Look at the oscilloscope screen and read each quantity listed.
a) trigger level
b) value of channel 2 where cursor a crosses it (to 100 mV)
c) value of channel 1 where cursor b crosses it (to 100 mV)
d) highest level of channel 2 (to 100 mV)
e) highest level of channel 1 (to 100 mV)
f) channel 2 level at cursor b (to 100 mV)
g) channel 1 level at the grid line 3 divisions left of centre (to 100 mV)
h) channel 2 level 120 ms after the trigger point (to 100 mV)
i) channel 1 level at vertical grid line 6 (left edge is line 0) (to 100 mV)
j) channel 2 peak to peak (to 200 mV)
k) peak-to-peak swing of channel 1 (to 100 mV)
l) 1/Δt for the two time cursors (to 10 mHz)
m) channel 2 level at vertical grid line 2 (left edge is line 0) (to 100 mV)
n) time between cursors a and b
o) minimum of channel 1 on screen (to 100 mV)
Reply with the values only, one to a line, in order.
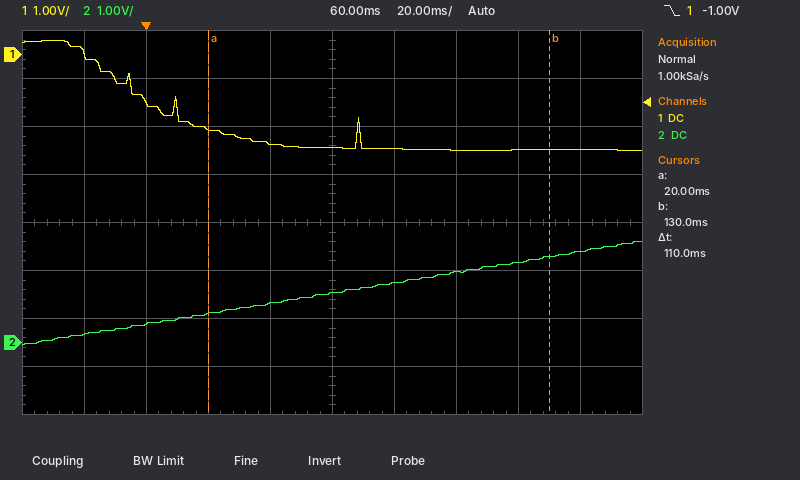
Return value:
-1.00 V
600 mV
-2.0 V
2.1 V
300 mV
1.8 V
-1.0 V
1.7 V
-2.0 V
2.2 V
2.3 V
9.09 Hz
400 mV
110 ms
-2.0 V
